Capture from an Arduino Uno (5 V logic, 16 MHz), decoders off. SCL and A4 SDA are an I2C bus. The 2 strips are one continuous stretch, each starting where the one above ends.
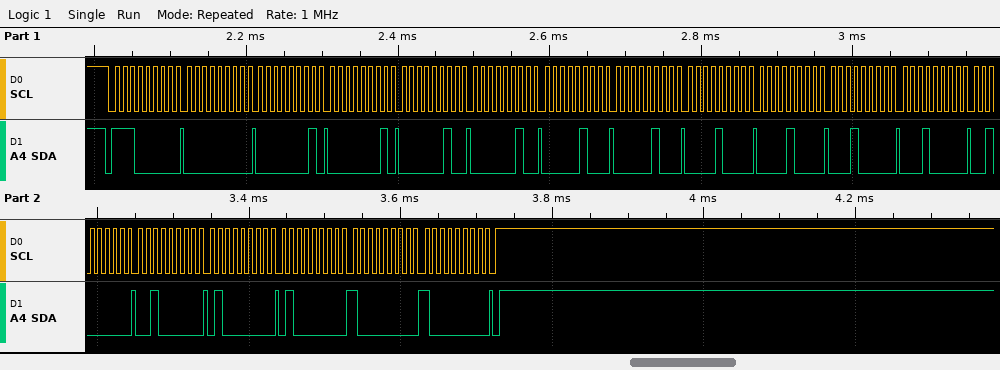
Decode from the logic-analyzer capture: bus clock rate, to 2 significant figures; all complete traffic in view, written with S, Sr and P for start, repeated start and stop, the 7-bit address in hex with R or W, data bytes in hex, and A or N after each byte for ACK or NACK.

100 kHz
S 70W A 00 A 01 A 01 A 02 A 02 A 04 A 04 A 08 A 08 A 10 A 10 A 20 A 20 A 40 A 40 A 80 A 80 A P
